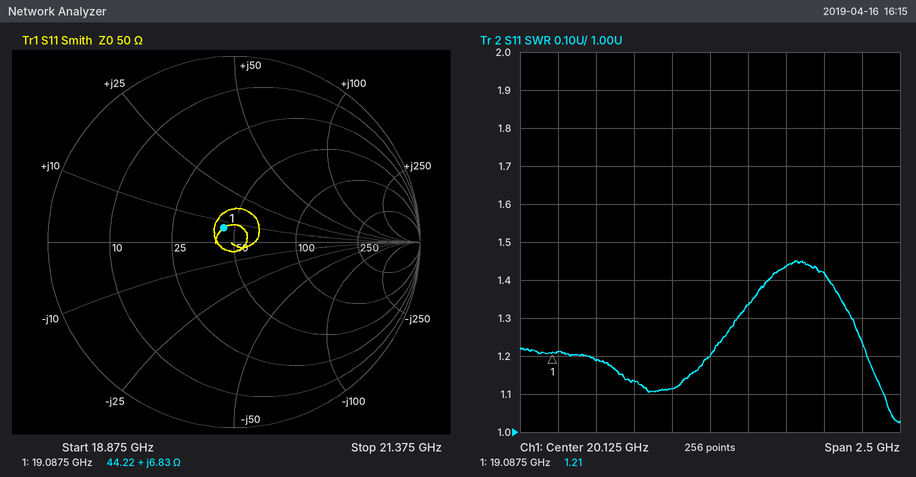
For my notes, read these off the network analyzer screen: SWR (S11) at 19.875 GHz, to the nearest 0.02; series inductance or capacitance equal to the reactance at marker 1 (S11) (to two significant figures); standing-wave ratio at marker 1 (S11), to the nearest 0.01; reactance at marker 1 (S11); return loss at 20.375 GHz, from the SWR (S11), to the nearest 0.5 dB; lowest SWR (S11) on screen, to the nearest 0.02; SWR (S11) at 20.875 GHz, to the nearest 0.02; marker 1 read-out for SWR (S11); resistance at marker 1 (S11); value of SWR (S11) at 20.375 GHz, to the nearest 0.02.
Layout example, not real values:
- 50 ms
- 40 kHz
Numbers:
- 1.12
- 57 pH
- 1.21
- +6.83 Ω
- 17.0 dB
- 1.02
- 1.42
- 1.21
- 44.22 Ω
- 1.34
